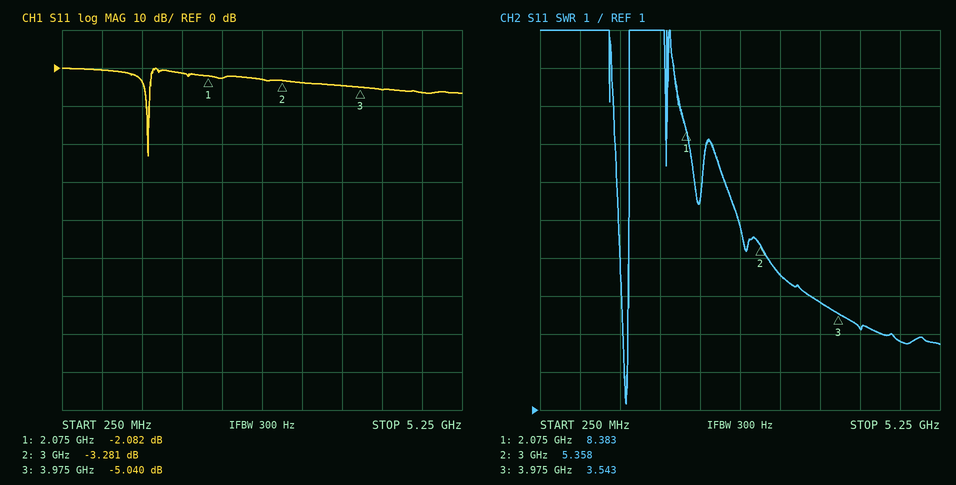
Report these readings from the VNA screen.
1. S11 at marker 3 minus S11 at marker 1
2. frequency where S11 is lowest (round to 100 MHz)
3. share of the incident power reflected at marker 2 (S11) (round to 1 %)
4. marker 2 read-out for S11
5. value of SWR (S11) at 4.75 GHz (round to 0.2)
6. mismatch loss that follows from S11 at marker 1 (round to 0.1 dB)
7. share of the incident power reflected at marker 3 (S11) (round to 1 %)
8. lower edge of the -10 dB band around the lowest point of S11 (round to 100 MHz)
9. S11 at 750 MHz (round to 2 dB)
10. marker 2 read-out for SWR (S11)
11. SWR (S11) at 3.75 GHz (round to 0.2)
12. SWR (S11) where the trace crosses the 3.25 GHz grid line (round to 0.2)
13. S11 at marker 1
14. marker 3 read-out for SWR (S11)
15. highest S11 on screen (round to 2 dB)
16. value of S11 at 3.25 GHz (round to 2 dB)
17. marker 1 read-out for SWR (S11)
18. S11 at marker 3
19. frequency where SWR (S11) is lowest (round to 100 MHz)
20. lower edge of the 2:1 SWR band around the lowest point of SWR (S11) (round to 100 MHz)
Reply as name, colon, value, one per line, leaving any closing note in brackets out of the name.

S11 at marker 3 minus S11 at marker 1: -2.958 dB
frequency where S11 is lowest: 1.3 GHz
share of the incident power reflected at marker 2 (S11): 47 %
marker 2 read-out for S11: -3.281 dB
value of SWR (S11) at 4.75 GHz: 2.8
mismatch loss that follows from S11 at marker 1: 4.2 dB
share of the incident power reflected at marker 3 (S11): 31 %
lower edge of the -10 dB band around the lowest point of S11: 1.3 GHz
S11 at 750 MHz: 0 dB
marker 2 read-out for SWR: 5.358
SWR (S11) at 3.75 GHz: 3.8
SWR (S11) where the trace crosses the 3.25 GHz grid line: 4.6
S11 at marker 1: -2.082 dB
marker 3 read-out for SWR: 3.543
highest S11 on screen: 0 dB
value of S11 at 3.25 GHz: -4 dB
marker 1 read-out for SWR: 8.383
S11 at marker 3: -5.040 dB
frequency where SWR (S11) is lowest: 1.3 GHz
lower edge of the 2:1 SWR band around the lowest point of SWR (S11): 1.3 GHz
